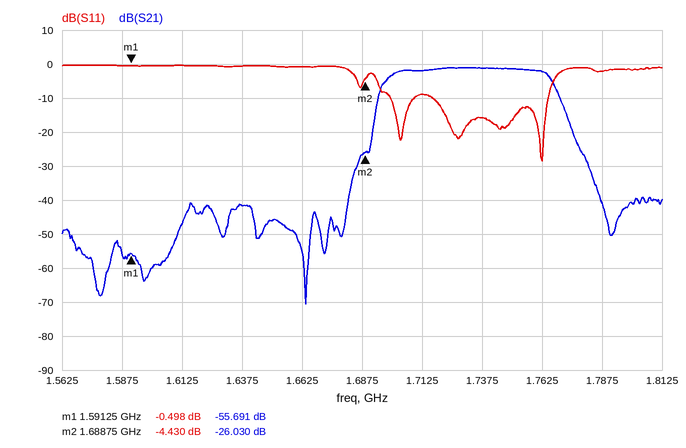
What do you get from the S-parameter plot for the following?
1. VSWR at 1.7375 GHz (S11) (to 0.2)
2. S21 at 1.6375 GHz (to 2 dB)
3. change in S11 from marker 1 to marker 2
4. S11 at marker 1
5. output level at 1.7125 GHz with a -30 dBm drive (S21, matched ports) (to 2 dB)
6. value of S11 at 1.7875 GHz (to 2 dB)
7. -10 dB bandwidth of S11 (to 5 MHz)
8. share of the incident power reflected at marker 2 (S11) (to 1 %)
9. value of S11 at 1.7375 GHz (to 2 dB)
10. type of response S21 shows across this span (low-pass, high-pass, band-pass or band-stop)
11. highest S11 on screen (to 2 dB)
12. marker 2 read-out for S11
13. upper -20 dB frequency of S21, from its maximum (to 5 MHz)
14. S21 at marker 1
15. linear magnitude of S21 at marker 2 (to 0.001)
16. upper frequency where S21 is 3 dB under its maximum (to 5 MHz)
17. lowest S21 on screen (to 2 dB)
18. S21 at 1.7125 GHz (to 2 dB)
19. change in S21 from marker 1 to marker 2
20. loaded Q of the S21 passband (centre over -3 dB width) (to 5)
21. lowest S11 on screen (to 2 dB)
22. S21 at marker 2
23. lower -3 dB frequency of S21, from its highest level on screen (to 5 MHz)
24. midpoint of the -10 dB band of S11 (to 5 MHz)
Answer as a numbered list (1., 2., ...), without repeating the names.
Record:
1. 1.4
2. -42 dB
3. -3.932 dB
4. -0.498 dB
5. -32 dBm
6. -2 dB
7. 50 MHz
8. 36 %
9. -16 dB
10. band-pass
11. 0 dB
12. -4.430 dB
13. 1.775 GHz
14. -55.691 dB
15. 0.050
16. 1.765 GHz
17. -70 dB
18. -2 dB
19. 29.661 dB
20. 25
21. -28 dB
22. -26.030 dB
23. 1.700 GHz
24. 1.740 GHz
